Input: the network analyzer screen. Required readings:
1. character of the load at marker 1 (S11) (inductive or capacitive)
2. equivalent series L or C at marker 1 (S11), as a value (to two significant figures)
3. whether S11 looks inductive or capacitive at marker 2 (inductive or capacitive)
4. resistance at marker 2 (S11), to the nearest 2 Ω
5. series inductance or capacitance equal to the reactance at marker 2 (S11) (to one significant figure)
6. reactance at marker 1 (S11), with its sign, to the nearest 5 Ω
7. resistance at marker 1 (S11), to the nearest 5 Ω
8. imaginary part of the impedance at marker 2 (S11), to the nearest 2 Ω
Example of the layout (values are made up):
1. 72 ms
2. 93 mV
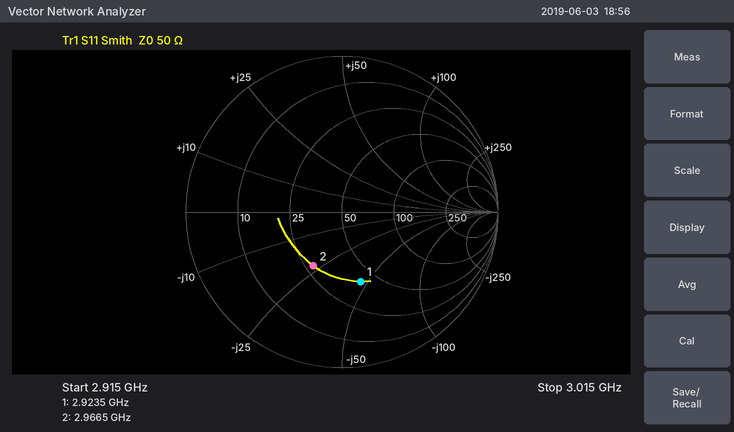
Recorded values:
1. capacitive
2. 1.2 pF
3. capacitive
4. 28 Ω
5. 2 pF
6. -45 Ω
7. 40 Ω
8. -22 Ω
